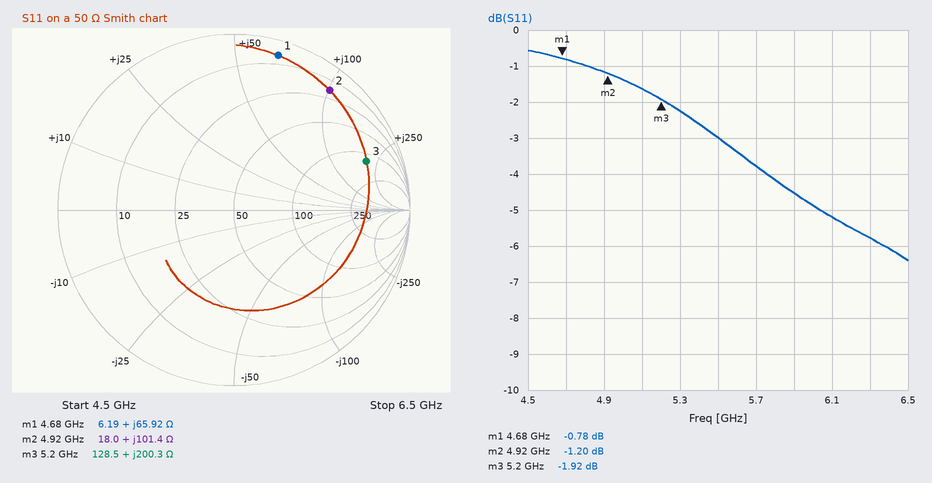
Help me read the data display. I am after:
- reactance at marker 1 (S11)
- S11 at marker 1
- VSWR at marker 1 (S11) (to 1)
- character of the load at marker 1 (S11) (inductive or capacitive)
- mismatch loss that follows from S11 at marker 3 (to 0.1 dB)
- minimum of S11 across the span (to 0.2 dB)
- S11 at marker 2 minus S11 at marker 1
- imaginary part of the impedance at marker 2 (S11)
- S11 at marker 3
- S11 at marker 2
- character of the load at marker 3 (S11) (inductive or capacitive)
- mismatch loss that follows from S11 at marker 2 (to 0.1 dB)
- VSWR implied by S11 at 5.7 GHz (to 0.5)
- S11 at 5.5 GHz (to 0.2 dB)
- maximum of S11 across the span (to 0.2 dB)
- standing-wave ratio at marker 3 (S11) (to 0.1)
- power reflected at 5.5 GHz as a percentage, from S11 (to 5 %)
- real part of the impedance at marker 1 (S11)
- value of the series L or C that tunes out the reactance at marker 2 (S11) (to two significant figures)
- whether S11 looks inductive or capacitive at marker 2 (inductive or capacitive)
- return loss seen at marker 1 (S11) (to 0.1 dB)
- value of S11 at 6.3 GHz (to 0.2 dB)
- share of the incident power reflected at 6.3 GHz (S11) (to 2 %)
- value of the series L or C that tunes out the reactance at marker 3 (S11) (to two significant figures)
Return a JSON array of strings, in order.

["+65.92 Ω", "-0.78 dB", "22", "inductive", "4.5 dB", "-6.4 dB", "-0.42 dB", "+101.4 Ω", "-1.92 dB", "-1.20 dB", "inductive", "6.2 dB", "4.5", "-3.0 dB", "-0.6 dB", "9.1", "50 %", "6.19 Ω", "320 fF", "inductive", "0.8 dB", "-5.8 dB", "26 %", "150 fF"]
